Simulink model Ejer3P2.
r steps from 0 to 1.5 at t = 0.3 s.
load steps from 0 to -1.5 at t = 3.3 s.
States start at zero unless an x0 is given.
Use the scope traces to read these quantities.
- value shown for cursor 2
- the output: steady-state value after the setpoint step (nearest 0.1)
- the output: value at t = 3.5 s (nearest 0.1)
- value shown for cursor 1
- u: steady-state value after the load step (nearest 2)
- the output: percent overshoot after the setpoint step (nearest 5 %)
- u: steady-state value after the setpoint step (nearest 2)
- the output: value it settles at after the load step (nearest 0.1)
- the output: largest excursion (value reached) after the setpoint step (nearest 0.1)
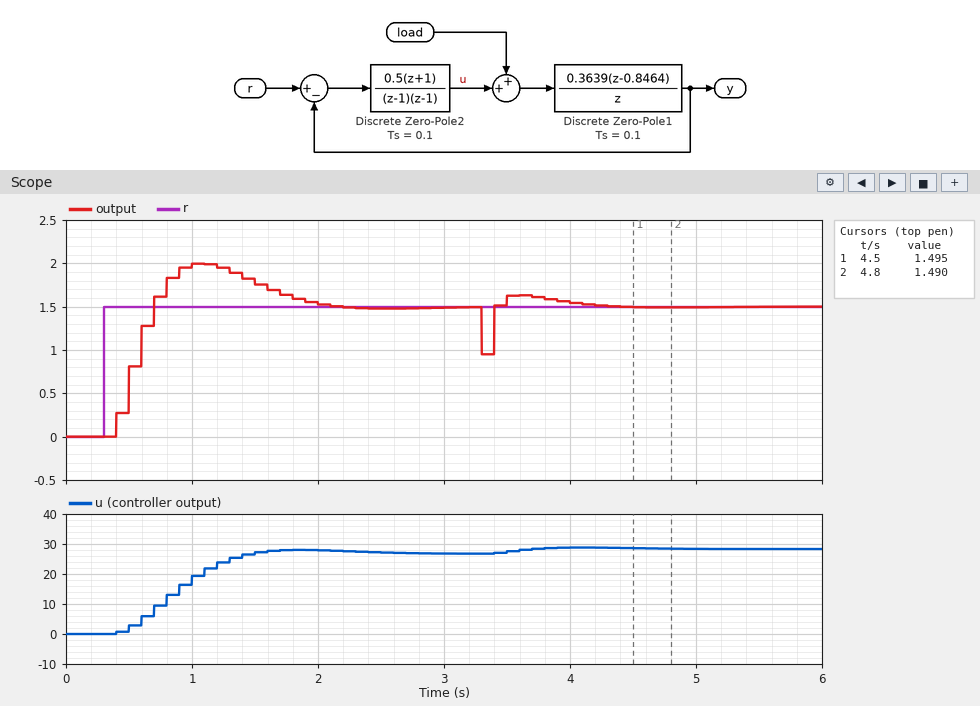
1.490
1.5
1.6
1.495
28
35 %
26
1.5
2.0
